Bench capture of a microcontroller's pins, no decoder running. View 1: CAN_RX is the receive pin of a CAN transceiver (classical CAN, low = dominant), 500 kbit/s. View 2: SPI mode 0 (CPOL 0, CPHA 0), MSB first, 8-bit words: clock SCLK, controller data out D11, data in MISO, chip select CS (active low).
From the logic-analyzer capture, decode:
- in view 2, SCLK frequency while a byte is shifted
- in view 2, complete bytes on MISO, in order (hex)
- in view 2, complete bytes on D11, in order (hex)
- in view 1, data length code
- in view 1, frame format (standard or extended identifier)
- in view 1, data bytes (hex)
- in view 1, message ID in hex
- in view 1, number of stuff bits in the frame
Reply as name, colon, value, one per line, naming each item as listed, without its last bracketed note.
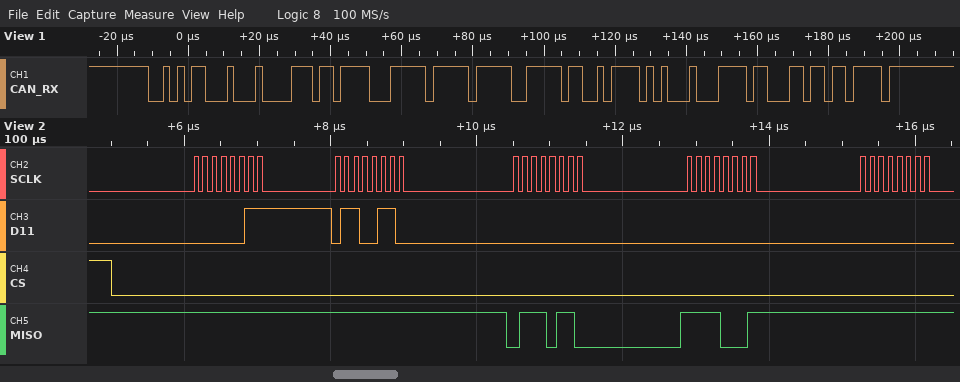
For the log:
in view 2, SCLK frequency while a byte is shifted: 8 MHz
in view 2, complete bytes on MISO, in order: FF FF 76 F1 FF
in view 2, complete bytes on D11, in order: 03 66 00 00 00
in view 1, data length code: 8
in view 1, frame format: standard
in view 1, data bytes: 76 F1 FF FD FC BD 44 7B
in view 1, message ID in hex: 0x2B1
in view 1, number of stuff bits in the frame: 4
